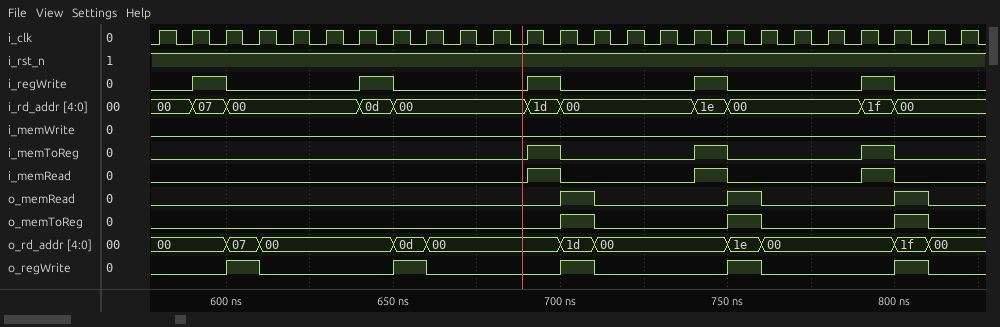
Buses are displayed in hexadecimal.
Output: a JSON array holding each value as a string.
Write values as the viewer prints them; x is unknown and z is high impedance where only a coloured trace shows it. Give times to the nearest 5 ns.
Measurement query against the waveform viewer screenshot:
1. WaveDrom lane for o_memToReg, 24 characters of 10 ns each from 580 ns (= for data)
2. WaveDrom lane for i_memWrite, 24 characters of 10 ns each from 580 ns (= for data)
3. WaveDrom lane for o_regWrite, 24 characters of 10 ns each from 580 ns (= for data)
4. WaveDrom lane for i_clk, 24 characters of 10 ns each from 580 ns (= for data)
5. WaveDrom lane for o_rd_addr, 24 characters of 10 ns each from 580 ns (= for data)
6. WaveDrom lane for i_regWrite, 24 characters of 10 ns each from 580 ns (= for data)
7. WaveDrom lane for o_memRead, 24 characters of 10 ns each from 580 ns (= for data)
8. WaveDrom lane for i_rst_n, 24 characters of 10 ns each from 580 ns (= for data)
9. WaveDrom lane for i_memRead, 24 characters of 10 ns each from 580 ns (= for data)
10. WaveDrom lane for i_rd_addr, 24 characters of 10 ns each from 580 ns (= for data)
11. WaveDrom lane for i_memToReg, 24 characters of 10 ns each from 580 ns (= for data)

["{name: 'o_memToReg', wave: '0...........10...10...10'}", "{name: 'i_memWrite', wave: '0.......................'}", "{name: 'o_regWrite', wave: '0.10...10...10...10...10'}", "{name: 'i_clk', wave: 'p.......................'}", "{name: 'o_rd_addr', wave: '=.==...==...==...==...==', data: '00 07 00 0d 00 1d 00 1e 00 1f 00'}", "{name: 'i_regWrite', wave: '010...10...10...10...10.'}", "{name: 'o_memRead', wave: '0...........10...10...10'}", "{name: 'i_rst_n', wave: '1.......................'}", "{name: 'i_memRead', wave: '0..........10...10...10.'}", "{name: 'i_rd_addr', wave: '===...==...==...==...==.', data: '00 07 00 0d 00 1d 00 1e 00 1f 00'}", "{name: 'i_memToReg', wave: '0..........10...10...10.'}"]
